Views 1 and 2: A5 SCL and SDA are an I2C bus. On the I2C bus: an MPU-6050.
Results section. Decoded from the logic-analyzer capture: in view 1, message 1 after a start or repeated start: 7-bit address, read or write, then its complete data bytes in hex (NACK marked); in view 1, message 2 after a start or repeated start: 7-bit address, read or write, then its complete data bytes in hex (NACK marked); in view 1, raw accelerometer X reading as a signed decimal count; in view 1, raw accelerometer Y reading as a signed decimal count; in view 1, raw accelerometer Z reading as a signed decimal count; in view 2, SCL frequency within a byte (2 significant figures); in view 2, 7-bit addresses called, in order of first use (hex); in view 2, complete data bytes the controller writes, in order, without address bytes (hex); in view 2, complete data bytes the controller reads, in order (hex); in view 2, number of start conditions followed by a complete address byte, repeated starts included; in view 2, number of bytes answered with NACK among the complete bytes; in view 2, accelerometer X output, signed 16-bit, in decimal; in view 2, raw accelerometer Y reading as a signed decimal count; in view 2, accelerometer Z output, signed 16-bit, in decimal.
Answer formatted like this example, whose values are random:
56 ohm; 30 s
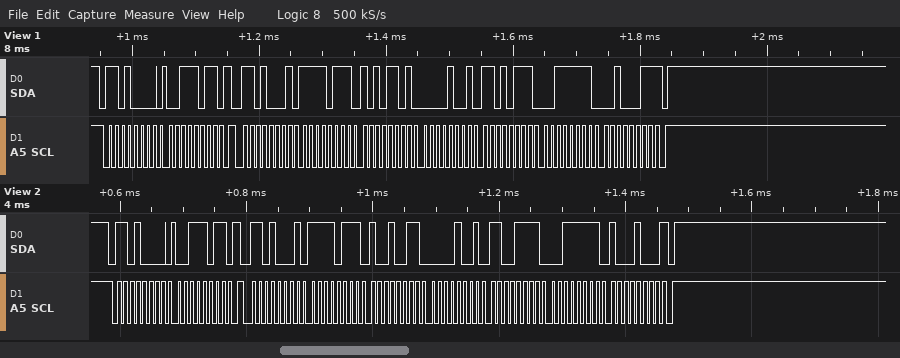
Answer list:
0x68 write: 3B; 0x68 read: F7 AD 09 D7 3F 23 NACK; -2131; 2519; 16163; 100 kHz; 0x68; 3B; F7 93 09 CF 3F 88; 2; 1; -2157; 2511; 16264
